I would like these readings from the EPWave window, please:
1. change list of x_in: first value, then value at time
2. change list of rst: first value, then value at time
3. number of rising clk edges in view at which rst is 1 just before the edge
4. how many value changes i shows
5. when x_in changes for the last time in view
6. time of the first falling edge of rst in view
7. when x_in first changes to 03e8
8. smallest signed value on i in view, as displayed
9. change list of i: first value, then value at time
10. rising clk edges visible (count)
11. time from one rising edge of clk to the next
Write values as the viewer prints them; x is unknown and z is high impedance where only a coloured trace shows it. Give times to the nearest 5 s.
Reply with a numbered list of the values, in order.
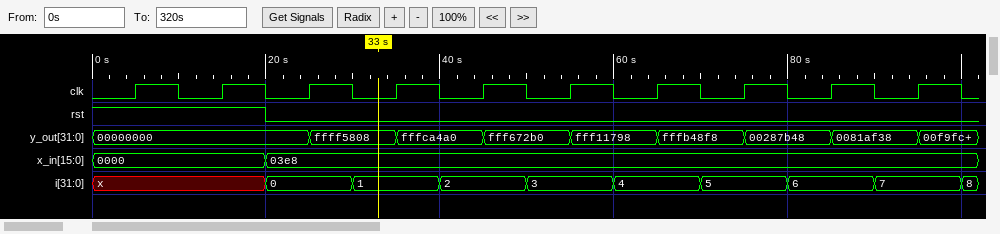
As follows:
1. 0000, 03e8 at 20 s
2. 1, 0 at 20 s
3. 2
4. 9
5. 20 s
6. 20 s
7. 20 s
8. 0
9. x, 0 at 20 s, 1 at 30 s, 2 at 40 s, 3 at 50 s, 4 at 60 s, 5 at 70 s, 6 at 80 s, 7 at 90 s, 8 at 100 s
10. 10
11. 10 s
